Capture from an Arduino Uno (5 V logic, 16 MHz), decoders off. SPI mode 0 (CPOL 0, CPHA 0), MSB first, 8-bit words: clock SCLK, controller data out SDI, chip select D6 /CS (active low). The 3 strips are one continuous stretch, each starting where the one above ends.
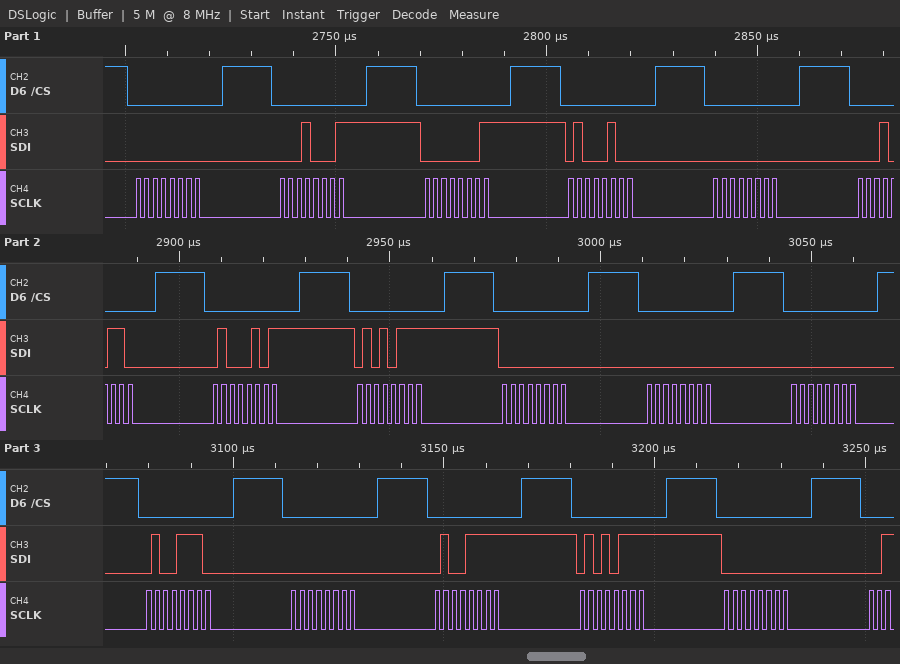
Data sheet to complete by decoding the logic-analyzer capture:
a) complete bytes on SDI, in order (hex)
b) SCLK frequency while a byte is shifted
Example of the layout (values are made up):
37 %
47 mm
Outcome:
00 11 01 44 00 16 45 57 00 00 00 4E 00 4F 57 00
500 kHz
